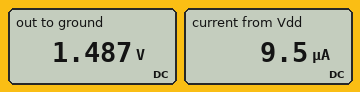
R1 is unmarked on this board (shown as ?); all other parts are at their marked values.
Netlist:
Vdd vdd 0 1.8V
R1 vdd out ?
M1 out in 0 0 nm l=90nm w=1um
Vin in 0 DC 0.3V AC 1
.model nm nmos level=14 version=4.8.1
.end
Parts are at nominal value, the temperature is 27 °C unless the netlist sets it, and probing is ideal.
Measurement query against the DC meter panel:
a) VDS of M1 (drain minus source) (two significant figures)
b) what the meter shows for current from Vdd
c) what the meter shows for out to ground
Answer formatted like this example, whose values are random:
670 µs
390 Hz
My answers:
1.5 V
9.5 µA
1.487 V
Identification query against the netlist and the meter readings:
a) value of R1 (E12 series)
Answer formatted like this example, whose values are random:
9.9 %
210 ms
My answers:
33 kΩ
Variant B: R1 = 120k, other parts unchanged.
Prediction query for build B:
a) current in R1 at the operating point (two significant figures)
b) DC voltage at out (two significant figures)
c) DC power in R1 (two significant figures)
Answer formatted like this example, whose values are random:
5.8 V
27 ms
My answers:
5.8 µA
1.1 V
4.1 µW
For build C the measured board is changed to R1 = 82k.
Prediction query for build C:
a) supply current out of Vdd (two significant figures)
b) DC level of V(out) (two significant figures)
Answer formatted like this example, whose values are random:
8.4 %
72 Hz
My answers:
6.9 µA
1.2 V
